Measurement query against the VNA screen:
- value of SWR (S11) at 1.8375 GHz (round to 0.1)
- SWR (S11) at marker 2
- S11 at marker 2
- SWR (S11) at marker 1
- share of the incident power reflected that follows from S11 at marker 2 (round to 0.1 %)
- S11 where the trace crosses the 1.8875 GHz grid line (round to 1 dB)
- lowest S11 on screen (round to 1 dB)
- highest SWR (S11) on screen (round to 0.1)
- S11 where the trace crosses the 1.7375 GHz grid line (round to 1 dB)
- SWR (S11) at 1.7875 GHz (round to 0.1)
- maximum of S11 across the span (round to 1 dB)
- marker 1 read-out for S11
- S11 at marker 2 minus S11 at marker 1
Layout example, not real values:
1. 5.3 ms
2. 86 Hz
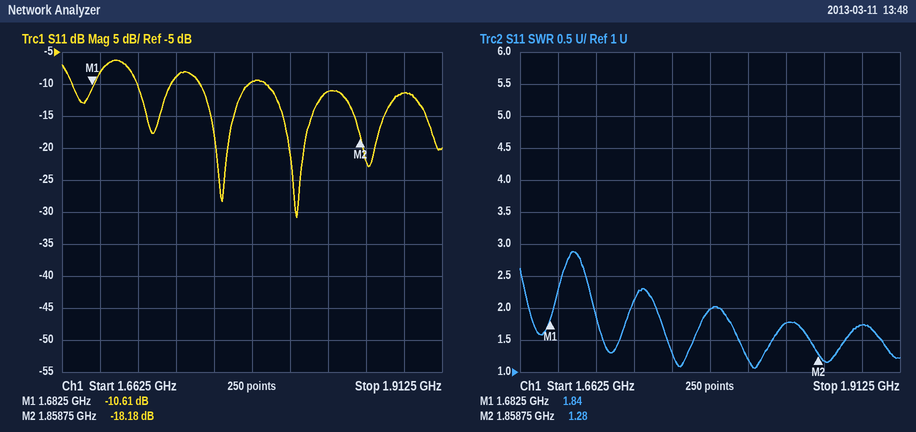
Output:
1. 1.8
2. 1.28
3. -18.18 dB
4. 1.84
5. 1.5 %
6. -11 dB
7. -31 dB
8. 2.9
9. -9 dB
10. 2.0
11. -6 dB
12. -10.61 dB
13. -7.57 dB
